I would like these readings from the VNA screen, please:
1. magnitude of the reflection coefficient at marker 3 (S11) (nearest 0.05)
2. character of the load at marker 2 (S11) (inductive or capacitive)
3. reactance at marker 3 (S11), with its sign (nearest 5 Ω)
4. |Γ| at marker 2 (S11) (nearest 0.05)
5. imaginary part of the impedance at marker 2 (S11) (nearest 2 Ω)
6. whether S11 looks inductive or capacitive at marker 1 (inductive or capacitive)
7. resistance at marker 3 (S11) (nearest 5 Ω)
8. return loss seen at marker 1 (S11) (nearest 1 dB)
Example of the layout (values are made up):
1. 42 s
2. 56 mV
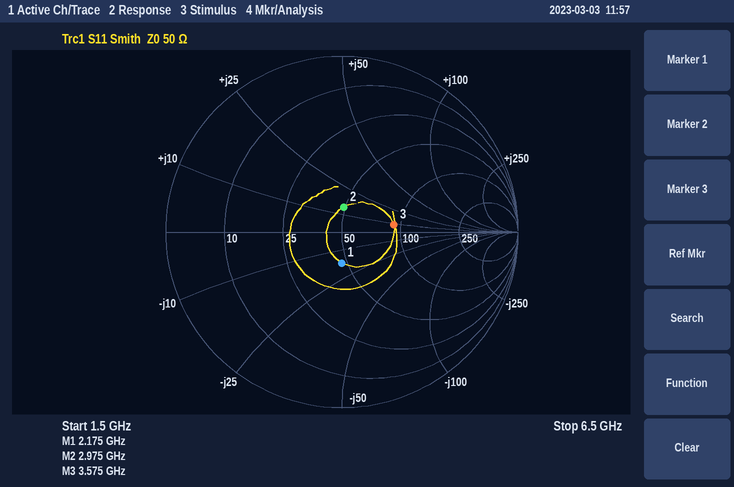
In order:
1. 0.30
2. inductive
3. +10 Ω
4. 0.15
5. +14 Ω
6. capacitive
7. 90 Ω
8. 15 dB
